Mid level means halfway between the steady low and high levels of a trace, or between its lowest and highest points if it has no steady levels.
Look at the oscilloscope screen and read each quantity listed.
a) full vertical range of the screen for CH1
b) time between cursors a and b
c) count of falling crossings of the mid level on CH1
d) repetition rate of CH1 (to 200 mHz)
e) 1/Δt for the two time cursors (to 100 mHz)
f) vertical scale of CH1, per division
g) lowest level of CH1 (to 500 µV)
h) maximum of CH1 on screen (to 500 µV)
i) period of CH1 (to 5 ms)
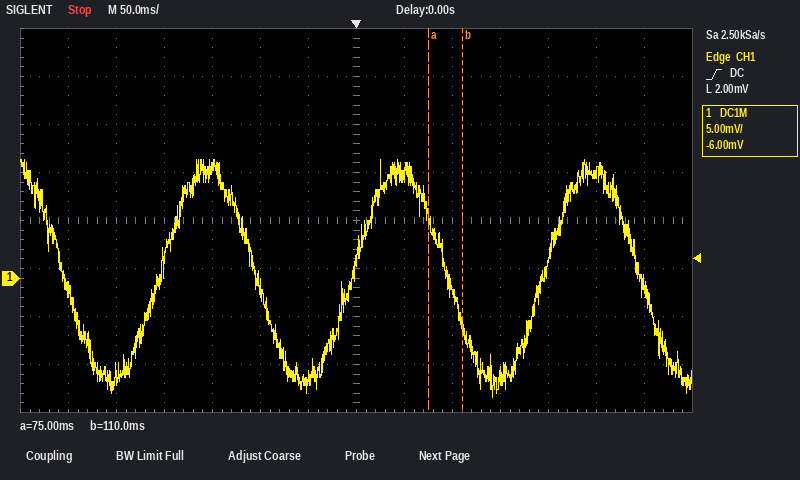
40 mV
35 ms
4
5.0 Hz
28.6 Hz
5 mV
-12.5 mV
12.5 mV
200 ms
